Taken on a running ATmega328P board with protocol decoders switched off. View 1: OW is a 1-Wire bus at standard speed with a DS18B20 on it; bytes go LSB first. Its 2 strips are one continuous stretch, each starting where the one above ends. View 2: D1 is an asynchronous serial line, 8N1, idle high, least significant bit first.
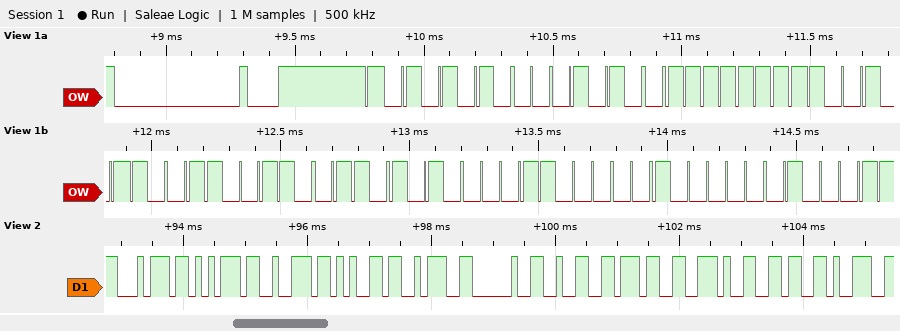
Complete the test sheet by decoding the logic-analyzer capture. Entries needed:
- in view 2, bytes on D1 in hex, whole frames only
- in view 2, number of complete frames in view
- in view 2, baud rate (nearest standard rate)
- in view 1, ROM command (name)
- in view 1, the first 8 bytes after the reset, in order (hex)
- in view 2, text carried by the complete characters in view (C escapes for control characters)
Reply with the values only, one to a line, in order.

74 75 72 65 3A 20 32 37 2E 36 39
11
9600 baud
Match ROM
55 28 FF 69 66 56 18 04
"ture: 27.69"
